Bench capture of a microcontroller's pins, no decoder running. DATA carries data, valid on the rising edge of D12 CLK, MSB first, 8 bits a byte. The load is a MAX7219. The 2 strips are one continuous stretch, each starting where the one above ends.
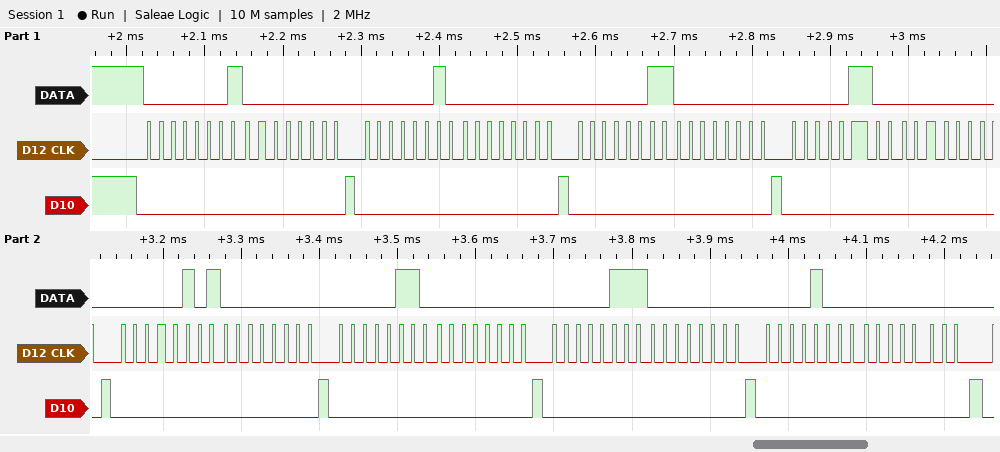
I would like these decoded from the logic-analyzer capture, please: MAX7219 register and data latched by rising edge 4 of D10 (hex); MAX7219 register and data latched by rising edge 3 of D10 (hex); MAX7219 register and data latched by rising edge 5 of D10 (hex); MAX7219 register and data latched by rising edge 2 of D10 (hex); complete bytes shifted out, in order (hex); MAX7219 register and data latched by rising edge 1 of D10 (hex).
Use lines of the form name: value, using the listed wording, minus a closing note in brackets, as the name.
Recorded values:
MAX7219 register and data latched by rising edge 4 of D10: register 0x4, data 0x00
MAX7219 register and data latched by rising edge 3 of D10: register 0x3, data 0x00
MAX7219 register and data latched by rising edge 5 of D10: register 0x5, data 0x00
MAX7219 register and data latched by rising edge 2 of D10: register 0x2, data 0x00
complete bytes shifted out, in order: 0x01 0x00 0x02 0x00 0x03 0x00 0x04 0x00 0x05 0x00 0x06 0x00 0x07 0x00 0x08 0x00
MAX7219 register and data latched by rising edge 1 of D10: register 0x1, data 0x00
